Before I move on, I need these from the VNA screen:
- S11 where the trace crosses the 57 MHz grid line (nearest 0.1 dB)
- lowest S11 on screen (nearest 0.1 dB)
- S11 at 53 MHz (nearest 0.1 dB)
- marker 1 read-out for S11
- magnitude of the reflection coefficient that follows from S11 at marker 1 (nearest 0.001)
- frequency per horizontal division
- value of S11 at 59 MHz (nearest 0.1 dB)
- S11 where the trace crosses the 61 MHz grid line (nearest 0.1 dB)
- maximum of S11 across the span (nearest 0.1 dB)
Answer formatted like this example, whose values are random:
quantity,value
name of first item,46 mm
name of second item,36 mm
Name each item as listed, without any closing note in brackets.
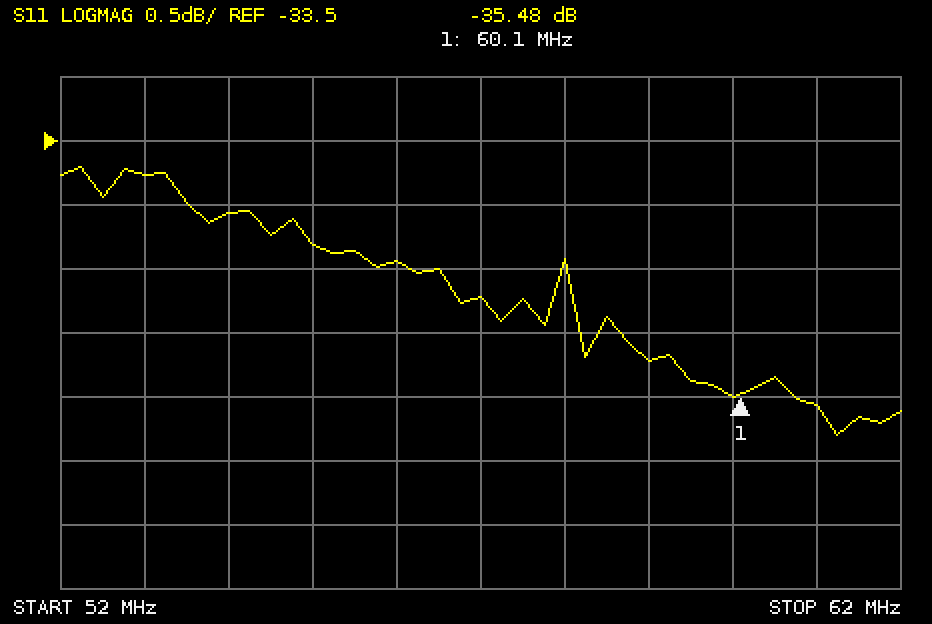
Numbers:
quantity,value
S11 where the trace crosses the 57 MHz grid line,-34.7 dB
lowest S11 on screen,-35.8 dB
S11 at 53 MHz,-33.8 dB
marker 1 read-out for S11,-35.48 dB
magnitude of the reflection coefficient that follows from S11 at marker 1,0.017
frequency per horizontal division,1 MHz
value of S11 at 59 MHz,-35.2 dB
S11 where the trace crosses the 61 MHz grid line,-35.6 dB
maximum of S11 across the span,-33.7 dB
